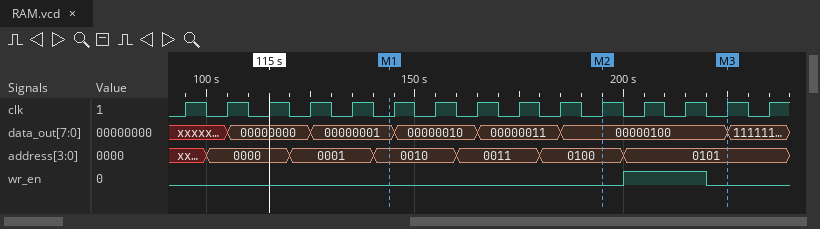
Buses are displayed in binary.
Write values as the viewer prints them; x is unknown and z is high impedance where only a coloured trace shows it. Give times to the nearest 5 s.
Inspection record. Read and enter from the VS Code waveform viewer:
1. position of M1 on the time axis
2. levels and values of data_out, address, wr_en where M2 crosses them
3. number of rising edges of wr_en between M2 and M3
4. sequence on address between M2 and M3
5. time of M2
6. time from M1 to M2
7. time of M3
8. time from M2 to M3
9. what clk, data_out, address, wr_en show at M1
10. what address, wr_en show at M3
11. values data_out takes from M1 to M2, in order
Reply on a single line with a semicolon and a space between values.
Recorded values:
145 s; data_out=00000100, address=0100, wr_en=0; 1; 0100, 0101; 195 s; 50 s; 225 s; 30 s; clk=0, data_out=00000001, address=0010, wr_en=0; address=0101, wr_en=0; 00000001, 00000010, 00000011, 00000100
